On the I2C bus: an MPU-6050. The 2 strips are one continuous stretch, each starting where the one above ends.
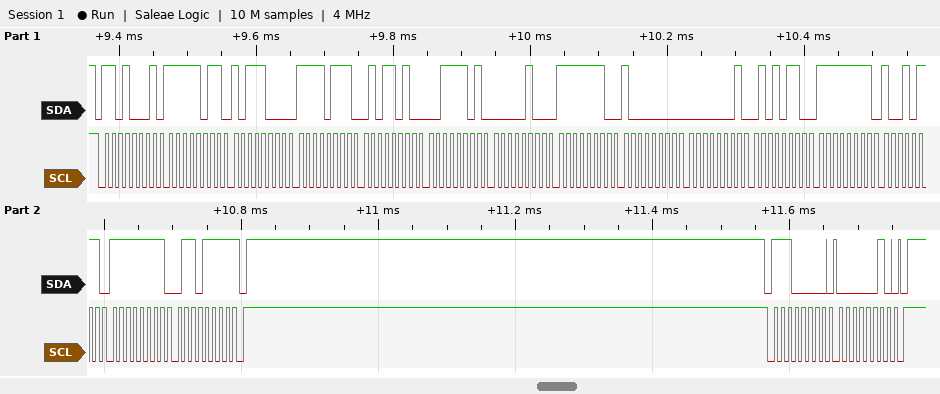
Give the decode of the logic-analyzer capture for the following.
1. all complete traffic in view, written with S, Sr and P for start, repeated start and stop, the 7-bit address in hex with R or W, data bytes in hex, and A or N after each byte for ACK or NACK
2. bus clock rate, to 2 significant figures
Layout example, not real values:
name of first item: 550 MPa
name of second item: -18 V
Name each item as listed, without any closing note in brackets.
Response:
all complete traffic in view, written with S, Sr and P for start, repeated start and stop, the 7-bit address in hex with R or W, data bytes in hex, and A or N after each byte for ACK or NACK: S 68R A FB A B8 A F7 A 5A A 3D A 04 A FE A 80 A 01 A 56 A FF A 97 A FF A 6F N P S 70W A 02 A P
bus clock rate, to 2 significant figures: 100 kHz
